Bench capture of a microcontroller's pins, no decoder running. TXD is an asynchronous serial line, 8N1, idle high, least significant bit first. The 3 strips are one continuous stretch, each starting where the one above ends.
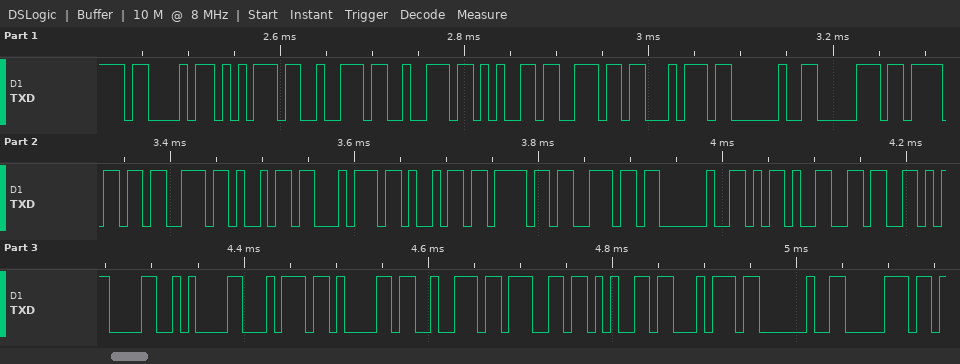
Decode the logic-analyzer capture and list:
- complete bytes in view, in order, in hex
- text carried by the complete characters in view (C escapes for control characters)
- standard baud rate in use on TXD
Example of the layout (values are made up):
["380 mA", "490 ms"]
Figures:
["0x43 0x75 0x72 0x72 0x65 0x6E 0x74 0x20 0x70 0x6F 0x73 0x69 0x74 0x69 0x6F 0x6E 0x20 0x2D 0x36 0x0D 0x0A 0x74 0x61 0x72 0x67 0x65 0x74 0x20 0x70", "\"Current position -6\\r\\ntarget p\"", "115200 baud"]
